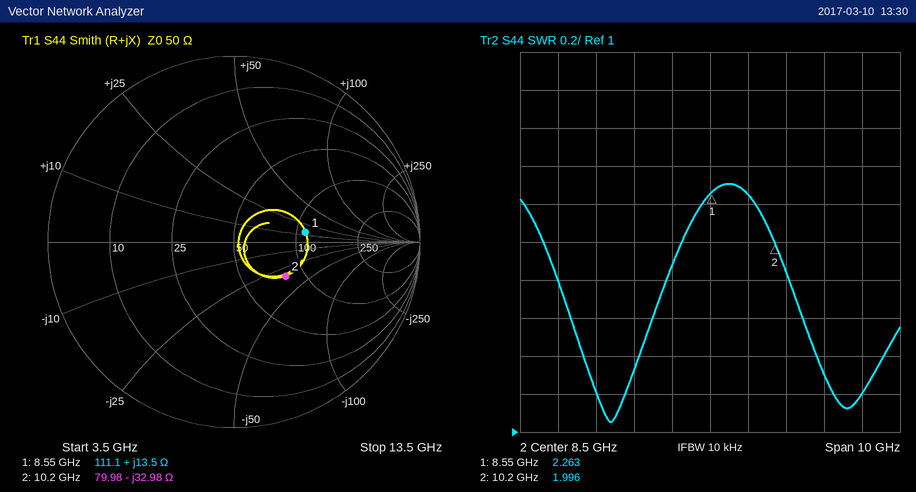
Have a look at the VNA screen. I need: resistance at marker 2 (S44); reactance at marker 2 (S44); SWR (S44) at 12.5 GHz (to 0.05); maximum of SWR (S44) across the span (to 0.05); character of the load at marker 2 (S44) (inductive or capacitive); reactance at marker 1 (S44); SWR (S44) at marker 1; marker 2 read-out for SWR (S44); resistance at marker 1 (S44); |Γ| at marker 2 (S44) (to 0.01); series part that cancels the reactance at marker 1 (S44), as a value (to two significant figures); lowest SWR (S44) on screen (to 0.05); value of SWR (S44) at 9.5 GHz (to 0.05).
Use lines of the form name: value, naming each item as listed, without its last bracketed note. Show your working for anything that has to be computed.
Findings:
resistance at marker 2: 79.98 Ω
reactance at marker 2: -32.98 Ω
SWR (S44) at 12.5 GHz: 1.20
maximum of SWR (S44) across the span: 2.30
character of the load at marker 2 (S44): capacitive
reactance at marker 1: +13.5 Ω
SWR (S44) at marker 1: 2.263
marker 2 read-out for SWR: 1.996
resistance at marker 1: 111.1 Ω
|Γ| at marker 2 (S44): 0.33
series part that cancels the reactance at marker 1 (S44), as a value: C = 1/(2π × 8.55 GHz × 13.5 Ω) ≈ 1.4 pF
lowest SWR (S44) on screen: 1.05
value of SWR (S44) at 9.5 GHz: 2.25
